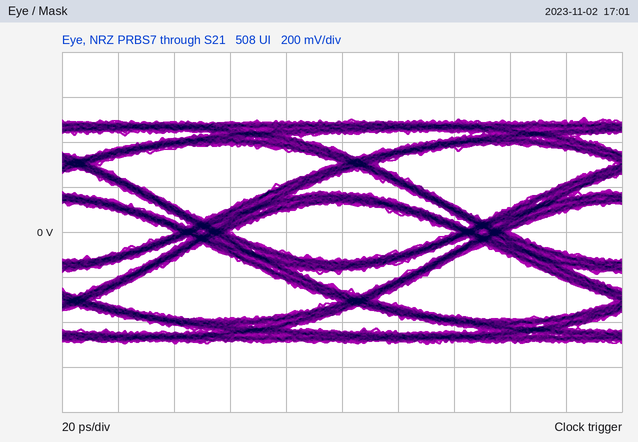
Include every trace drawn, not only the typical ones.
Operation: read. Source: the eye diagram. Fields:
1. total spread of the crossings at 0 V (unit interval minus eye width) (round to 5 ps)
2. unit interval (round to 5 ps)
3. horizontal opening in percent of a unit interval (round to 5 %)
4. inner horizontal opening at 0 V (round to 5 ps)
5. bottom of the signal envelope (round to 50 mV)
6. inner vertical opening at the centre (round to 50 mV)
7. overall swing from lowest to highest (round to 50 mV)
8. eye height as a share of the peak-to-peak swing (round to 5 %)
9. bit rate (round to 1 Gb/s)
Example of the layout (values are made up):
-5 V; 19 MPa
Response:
20 ps; 100 ps; 80 %; 80 ps; -500 mV; 250 mV; 1.00 V; 25 %; 10 Gb/s
